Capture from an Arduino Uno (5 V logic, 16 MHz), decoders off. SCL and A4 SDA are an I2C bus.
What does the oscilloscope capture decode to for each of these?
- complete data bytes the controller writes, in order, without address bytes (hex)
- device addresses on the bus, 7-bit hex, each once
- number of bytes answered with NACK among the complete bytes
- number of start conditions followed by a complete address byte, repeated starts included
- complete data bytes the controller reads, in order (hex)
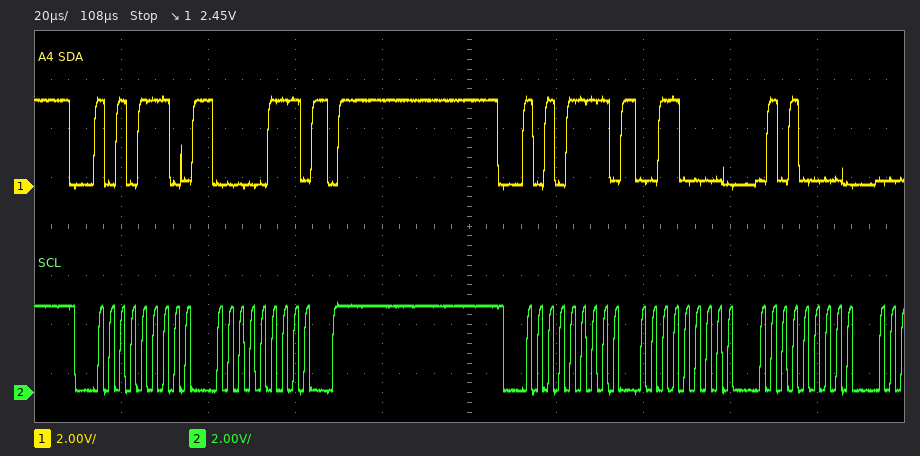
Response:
07
0x57
0
2
30 50
